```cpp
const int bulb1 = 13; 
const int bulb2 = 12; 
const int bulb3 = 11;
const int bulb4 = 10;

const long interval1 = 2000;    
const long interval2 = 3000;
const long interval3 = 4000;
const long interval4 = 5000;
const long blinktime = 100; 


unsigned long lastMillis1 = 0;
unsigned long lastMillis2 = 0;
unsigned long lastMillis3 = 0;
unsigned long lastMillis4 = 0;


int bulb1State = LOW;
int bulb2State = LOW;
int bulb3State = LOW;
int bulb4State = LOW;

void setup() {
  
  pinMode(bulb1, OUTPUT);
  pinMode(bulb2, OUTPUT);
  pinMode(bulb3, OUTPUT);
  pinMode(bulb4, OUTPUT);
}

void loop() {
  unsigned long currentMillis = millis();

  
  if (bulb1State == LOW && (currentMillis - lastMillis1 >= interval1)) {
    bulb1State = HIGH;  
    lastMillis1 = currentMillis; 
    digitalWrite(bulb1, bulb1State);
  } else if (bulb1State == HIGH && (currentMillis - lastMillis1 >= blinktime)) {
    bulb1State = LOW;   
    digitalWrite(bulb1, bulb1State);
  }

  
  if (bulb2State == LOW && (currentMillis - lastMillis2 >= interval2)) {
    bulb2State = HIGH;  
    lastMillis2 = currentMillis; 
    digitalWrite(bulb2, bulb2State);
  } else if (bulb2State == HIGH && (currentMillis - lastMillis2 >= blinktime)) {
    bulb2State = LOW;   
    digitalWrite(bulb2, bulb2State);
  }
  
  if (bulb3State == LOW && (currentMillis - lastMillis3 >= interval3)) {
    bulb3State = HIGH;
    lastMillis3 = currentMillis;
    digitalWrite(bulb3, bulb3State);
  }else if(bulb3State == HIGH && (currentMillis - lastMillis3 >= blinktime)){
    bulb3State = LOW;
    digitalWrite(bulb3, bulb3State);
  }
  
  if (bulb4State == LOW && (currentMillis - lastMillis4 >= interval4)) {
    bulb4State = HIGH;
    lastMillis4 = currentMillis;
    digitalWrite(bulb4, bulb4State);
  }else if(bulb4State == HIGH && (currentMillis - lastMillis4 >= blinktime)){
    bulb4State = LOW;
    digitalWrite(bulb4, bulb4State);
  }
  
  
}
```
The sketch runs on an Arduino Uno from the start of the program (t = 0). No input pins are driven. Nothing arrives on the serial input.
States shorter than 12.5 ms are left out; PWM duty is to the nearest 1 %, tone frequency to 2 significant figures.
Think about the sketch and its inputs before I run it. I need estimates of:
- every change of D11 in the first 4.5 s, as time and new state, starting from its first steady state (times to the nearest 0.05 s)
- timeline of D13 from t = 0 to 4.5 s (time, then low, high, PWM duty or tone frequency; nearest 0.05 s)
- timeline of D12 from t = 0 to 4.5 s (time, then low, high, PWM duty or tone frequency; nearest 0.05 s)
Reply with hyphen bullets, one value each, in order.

- 0 s low; 4 s high; 4.1 s low
- 0 s low; 2 s high; 2.1 s low; 4 s high; 4.1 s low
- 0 s low; 3 s high; 3.1 s low
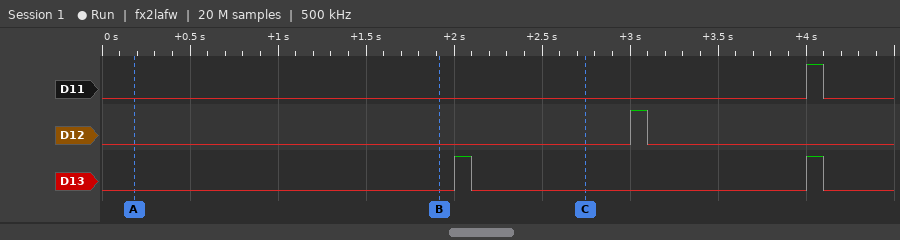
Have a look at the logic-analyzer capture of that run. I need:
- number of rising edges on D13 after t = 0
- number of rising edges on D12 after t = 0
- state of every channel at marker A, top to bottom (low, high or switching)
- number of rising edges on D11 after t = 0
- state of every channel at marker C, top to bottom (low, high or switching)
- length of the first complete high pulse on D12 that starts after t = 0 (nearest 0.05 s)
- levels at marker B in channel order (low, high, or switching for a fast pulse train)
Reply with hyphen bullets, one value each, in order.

- 2
- 1
- D11 low, D12 low, D13 low
- 1
- D11 low, D12 low, D13 low
- 0.10 s
- D11 low, D12 low, D13 low
